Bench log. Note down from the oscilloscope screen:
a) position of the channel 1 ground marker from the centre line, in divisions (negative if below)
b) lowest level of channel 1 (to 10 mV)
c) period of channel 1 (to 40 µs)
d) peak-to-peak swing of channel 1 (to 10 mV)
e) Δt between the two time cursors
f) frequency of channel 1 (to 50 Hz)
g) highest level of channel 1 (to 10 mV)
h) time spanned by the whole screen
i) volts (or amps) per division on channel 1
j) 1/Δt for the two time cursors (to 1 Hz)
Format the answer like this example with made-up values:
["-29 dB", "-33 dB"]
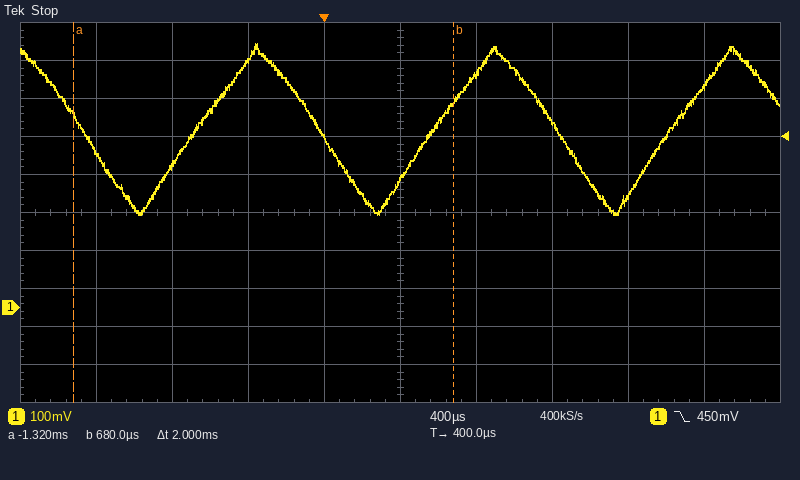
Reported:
["-2.5 div", "240 mV", "1.24 ms", "450 mV", "2 ms", "800 Hz", "690 mV", "4 ms", "100 mV", "500 Hz"]
